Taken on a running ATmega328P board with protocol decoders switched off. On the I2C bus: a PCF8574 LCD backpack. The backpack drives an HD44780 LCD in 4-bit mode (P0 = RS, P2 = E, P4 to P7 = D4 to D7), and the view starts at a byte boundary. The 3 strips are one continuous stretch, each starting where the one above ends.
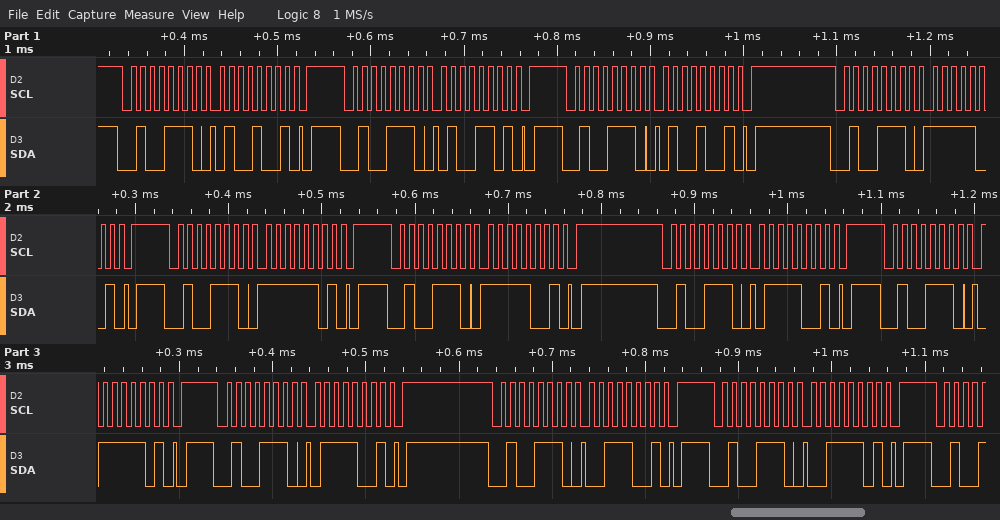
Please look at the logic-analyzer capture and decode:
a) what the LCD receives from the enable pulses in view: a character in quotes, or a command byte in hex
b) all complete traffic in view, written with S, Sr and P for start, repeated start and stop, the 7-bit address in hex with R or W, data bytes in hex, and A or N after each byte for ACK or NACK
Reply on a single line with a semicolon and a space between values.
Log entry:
'O'; S 27W A 49 A P S 27W A 4D A P S 27W A 49 A P S 27W A F9 A P S 27W A FD A P S 27W A F9 A P S 27W A 79 A P S 27W A 7D A P S 27W A 79 A P S 27W A 39 A P S 27W A 3D A P
